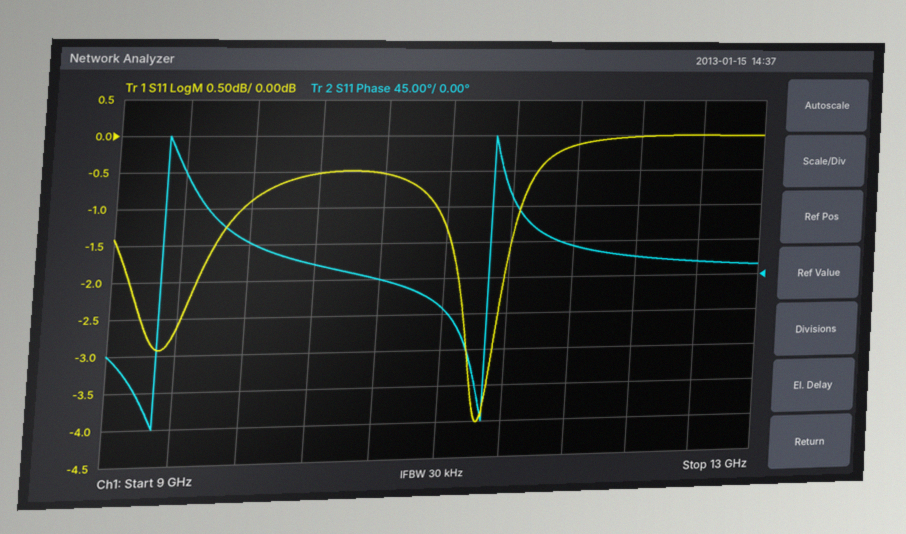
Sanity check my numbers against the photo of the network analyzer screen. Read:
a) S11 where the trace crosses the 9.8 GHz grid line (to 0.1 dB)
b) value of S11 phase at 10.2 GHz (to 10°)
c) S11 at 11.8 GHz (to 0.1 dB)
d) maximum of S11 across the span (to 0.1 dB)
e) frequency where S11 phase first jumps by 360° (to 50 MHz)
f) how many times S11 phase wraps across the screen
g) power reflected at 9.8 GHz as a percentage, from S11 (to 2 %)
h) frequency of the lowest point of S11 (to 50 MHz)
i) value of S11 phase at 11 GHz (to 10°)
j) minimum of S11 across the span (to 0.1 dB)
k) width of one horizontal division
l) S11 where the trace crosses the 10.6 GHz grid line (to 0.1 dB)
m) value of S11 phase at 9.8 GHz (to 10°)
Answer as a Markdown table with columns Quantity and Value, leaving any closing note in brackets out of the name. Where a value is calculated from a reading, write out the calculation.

| Quantity | Value |
|---|---|
| S11 where the trace crosses the 9.8 GHz grid line | -0.9 dB |
| value of S11 phase at 10.2 GHz | 20° |
| S11 at 11.8 GHz | -0.1 dB |
| maximum of S11 across the span | 0.0 dB |
| frequency where S11 phase first jumps by 360° | 9.30 GHz |
| how many times S11 phase wraps across the screen | 2 |
| power reflected at 9.8 GHz as a percentage, from S11 | 10^(-0.9/10) ≈ 81.3 %, so 82 % to the nearest 2 % |
| frequency of the lowest point of S11 | 11.25 GHz |
| value of S11 phase at 11 GHz | -40° |
| minimum of S11 across the span | -4.0 dB |
| width of one horizontal division | 400 MHz |
| S11 where the trace crosses the 10.6 GHz grid line | -0.5 dB |
| value of S11 phase at 9.8 GHz | 50° |
